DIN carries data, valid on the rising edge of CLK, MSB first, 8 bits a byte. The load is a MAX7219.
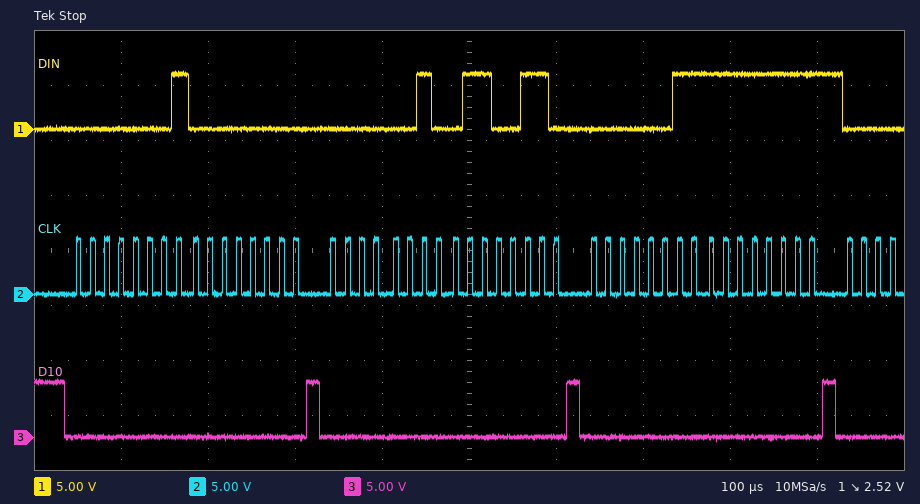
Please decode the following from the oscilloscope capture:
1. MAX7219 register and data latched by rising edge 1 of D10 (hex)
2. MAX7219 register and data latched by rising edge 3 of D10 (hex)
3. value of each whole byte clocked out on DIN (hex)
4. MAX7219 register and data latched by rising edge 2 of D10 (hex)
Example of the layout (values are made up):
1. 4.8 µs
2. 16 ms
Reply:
1. register 0x1, data 0x00
2. register 0x3, data 0xFF
3. 01 00 02 66 03 FF
4. register 0x2, data 0x66
